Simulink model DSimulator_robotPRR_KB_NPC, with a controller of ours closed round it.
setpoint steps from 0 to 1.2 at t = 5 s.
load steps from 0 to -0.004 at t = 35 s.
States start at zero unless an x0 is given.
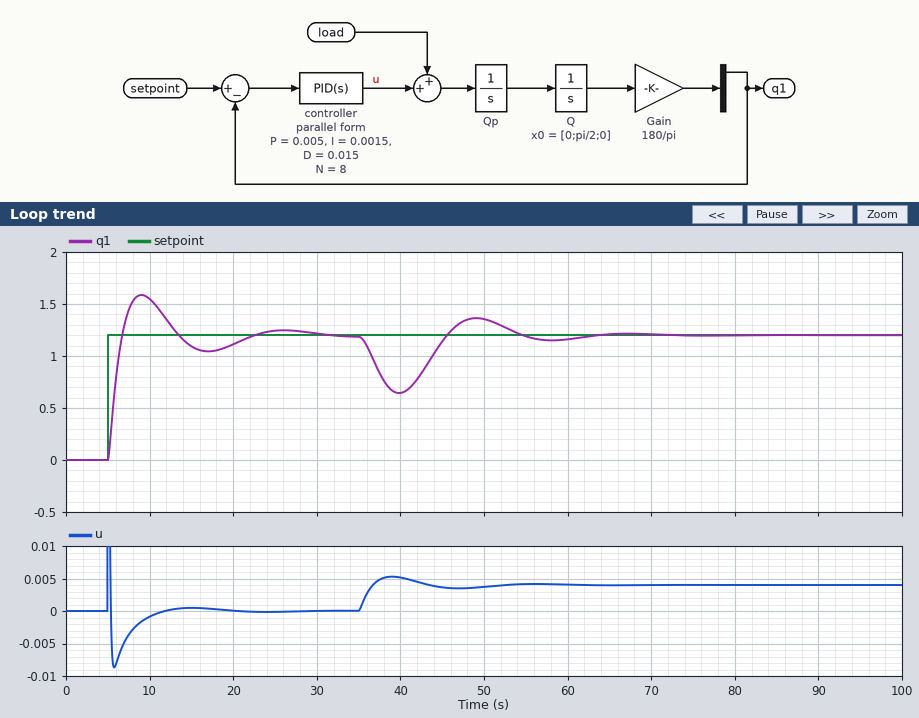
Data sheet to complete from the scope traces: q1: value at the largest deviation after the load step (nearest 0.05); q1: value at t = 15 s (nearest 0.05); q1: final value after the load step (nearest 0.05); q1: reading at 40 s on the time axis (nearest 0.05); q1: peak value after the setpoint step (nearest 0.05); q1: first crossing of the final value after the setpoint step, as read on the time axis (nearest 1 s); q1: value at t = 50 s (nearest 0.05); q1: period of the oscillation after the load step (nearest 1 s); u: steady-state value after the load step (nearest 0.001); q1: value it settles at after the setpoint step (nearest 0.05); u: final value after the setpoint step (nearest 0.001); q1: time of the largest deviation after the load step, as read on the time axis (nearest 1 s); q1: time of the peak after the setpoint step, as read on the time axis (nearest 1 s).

0.65
1.10
1.20
0.65
1.60
7 s
1.35
18 s
0.004
1.20
0.000
40 s
9 s
